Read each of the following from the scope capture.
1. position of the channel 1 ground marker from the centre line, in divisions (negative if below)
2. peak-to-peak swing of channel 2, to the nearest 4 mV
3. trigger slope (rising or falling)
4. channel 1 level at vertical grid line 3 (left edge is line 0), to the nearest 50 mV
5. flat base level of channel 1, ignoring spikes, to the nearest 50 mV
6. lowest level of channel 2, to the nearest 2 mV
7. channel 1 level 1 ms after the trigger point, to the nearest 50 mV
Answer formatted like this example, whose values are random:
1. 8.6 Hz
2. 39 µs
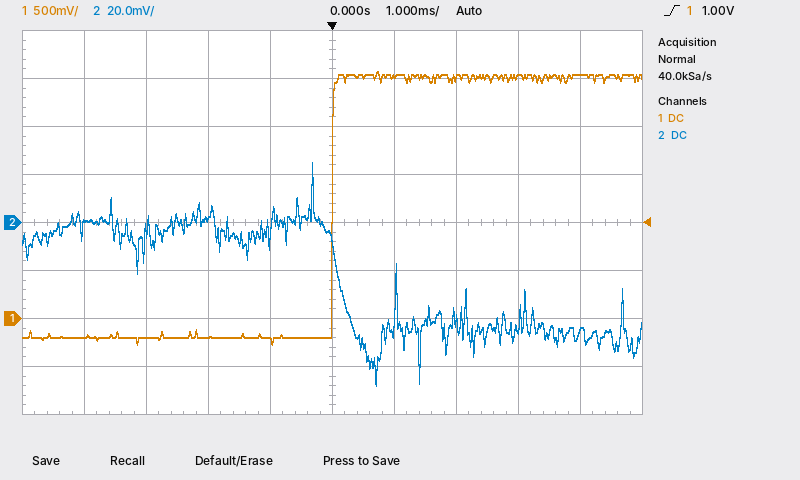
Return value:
1. -2.0 div
2. 92 mV
3. rising
4. -200 mV
5. -200 mV
6. -68 mV
7. 2.50 V
